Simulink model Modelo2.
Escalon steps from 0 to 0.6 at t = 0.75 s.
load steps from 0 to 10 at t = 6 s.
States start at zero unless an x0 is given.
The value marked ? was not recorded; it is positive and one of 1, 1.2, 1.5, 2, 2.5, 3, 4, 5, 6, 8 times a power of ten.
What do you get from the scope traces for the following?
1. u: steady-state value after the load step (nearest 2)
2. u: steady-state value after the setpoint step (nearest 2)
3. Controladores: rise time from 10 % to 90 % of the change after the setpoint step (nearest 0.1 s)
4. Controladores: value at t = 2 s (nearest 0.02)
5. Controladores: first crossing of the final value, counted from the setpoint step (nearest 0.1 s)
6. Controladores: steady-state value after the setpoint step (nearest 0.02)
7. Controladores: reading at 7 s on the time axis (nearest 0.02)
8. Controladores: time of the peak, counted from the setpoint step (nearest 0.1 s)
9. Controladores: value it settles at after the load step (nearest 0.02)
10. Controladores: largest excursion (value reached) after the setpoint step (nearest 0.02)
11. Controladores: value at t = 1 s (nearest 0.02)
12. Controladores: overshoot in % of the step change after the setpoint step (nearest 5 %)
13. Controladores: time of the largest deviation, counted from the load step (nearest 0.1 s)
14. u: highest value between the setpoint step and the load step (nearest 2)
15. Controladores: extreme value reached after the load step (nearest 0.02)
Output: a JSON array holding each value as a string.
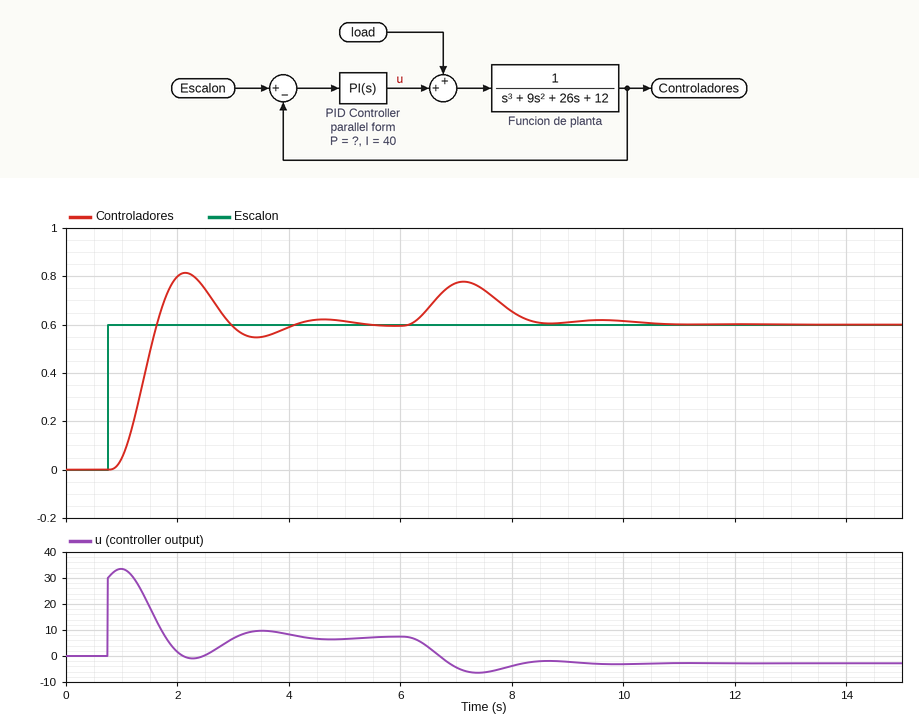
["-2", "8", "0.5 s", "0.80", "0.9 s", "0.60", "0.78", "1.4 s", "0.60", "0.82", "0.04", "35 %", "1.1 s", "34", "0.78"]
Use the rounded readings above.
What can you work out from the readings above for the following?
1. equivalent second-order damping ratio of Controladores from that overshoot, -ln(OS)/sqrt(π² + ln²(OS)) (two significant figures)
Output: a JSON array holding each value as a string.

["0.32"]
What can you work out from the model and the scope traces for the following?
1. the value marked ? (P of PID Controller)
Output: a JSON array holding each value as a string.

["50"]
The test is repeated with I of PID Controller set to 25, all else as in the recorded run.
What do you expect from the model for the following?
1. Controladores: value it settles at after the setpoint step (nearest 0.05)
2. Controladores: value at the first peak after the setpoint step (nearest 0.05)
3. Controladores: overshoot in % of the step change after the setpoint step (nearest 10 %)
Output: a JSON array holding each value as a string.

["0.60", "0.75", "20 %"]
